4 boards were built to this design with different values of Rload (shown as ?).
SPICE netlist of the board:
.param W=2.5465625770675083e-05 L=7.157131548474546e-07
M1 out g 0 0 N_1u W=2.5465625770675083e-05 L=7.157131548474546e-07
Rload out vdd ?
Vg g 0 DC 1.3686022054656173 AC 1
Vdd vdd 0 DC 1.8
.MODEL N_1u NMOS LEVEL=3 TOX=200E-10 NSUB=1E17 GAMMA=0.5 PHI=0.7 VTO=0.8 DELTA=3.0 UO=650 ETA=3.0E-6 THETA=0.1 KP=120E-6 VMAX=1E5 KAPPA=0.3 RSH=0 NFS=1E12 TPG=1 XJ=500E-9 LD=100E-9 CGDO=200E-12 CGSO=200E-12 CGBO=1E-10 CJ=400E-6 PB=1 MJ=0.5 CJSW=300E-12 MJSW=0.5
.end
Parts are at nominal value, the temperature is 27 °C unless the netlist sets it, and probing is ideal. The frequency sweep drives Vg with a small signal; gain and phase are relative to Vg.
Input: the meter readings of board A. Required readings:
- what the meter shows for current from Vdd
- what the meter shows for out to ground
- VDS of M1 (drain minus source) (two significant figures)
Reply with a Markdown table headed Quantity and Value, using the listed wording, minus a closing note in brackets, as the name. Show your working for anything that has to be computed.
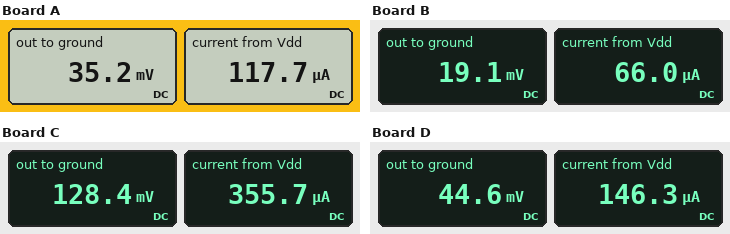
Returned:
| Quantity | Value |
|---|---|
| what the meter shows for current from Vdd | 117.7 µA |
| what the meter shows for out to ground | 35.2 mV |
| VDS of M1 (drain minus source) | 35.2 mV = 35 mV |
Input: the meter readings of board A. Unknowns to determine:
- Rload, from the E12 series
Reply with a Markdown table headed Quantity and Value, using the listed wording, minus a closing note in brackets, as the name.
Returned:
| Quantity | Value |
|---|---|
| Rload, from the E12 series | 15 kΩ |
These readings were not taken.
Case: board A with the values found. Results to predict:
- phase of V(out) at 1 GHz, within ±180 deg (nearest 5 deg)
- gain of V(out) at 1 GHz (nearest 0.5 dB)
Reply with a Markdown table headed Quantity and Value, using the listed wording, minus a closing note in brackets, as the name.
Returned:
| Quantity | Value |
|---|---|
| phase of V(out) at 1 GHz, within ±180 deg | 150 deg |
| gain of V(out) at 1 GHz | -24.0 dB |
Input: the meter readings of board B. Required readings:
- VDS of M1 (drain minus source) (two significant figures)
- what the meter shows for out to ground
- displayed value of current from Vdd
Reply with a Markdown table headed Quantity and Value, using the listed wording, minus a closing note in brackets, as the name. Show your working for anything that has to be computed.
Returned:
| Quantity | Value |
|---|---|
| VDS of M1 (drain minus source) | 19.1 mV = 19 mV |
| what the meter shows for out to ground | 19.1 mV |
| displayed value of current from Vdd | 66.0 µA |
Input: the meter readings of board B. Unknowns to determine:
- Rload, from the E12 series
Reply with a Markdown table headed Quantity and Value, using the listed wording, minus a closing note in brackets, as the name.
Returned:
| Quantity | Value |
|---|---|
| Rload, from the E12 series | 27 kΩ |
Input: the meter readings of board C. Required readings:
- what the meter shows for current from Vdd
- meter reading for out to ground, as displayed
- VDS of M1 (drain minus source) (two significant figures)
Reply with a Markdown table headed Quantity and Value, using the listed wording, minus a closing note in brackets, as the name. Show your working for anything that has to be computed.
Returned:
| Quantity | Value |
|---|---|
| what the meter shows for current from Vdd | 355.7 µA |
| meter reading for out to ground, as displayed | 128.4 mV |
| VDS of M1 (drain minus source) | 128.4 mV = 130 mV |
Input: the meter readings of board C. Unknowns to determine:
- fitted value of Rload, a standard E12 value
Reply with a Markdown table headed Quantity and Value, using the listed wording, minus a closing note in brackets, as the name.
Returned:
| Quantity | Value |
|---|---|
| fitted value of Rload, a standard E12 value | 4.7 kΩ |
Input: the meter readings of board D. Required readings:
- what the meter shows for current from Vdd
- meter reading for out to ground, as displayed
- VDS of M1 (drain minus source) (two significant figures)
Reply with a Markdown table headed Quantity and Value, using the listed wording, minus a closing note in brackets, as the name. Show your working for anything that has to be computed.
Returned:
| Quantity | Value |
|---|---|
| what the meter shows for current from Vdd | 146.3 µA |
| meter reading for out to ground, as displayed | 44.6 mV |
| VDS of M1 (drain minus source) | 44.6 mV = 45 mV |
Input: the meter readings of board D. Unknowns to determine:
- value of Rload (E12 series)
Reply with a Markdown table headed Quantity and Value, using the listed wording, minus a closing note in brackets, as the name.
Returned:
| Quantity | Value |
|---|---|
| value of Rload | 12 kΩ |
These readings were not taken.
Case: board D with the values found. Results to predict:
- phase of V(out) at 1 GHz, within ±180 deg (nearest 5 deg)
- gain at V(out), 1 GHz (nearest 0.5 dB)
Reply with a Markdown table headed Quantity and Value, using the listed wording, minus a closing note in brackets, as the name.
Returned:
| Quantity | Value |
|---|---|
| phase of V(out) at 1 GHz, within ±180 deg | 155 deg |
| gain at V(out), 1 GHz | -22.0 dB |
